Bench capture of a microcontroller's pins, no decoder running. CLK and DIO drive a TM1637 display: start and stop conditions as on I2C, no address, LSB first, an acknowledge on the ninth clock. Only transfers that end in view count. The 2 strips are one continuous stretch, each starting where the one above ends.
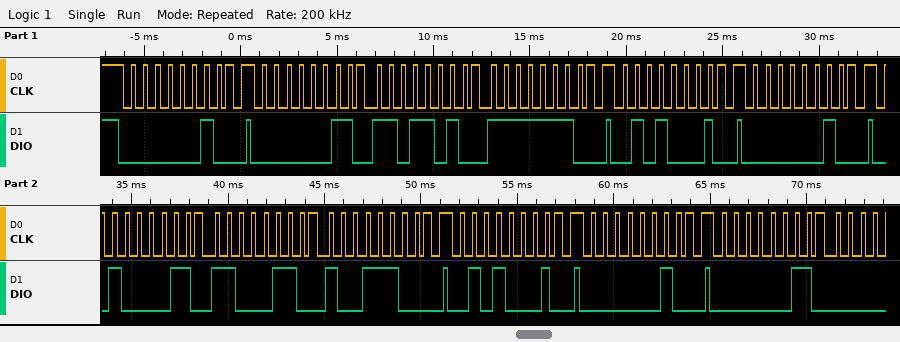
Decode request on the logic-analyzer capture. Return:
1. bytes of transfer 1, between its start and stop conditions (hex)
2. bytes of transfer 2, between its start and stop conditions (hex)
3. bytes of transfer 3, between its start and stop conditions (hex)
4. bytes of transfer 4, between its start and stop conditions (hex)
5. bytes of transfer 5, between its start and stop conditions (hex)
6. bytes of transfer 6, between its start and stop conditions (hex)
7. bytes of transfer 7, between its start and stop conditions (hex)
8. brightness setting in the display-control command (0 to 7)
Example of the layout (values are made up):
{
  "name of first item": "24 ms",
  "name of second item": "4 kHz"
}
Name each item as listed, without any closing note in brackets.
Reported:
{
  "bytes of transfer 1, between its start and stop conditions": "40",
  "bytes of transfer 2, between its start and stop conditions": "C0 5B 7F",
  "bytes of transfer 3, between its start and stop conditions": "8A",
  "bytes of transfer 4, between its start and stop conditions": "40",
  "bytes of transfer 5, between its start and stop conditions": "C2 63 39",
  "bytes of transfer 6, between its start and stop conditions": "8A",
  "bytes of transfer 7, between its start and stop conditions": "40",
  "brightness setting in the display-control command": "2"
}
